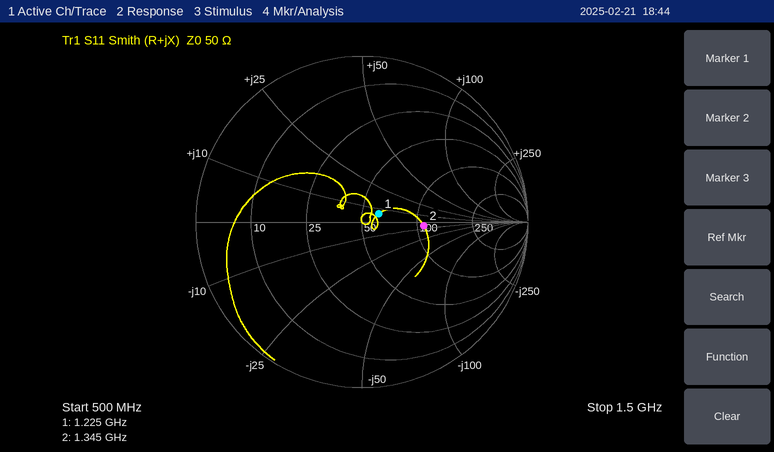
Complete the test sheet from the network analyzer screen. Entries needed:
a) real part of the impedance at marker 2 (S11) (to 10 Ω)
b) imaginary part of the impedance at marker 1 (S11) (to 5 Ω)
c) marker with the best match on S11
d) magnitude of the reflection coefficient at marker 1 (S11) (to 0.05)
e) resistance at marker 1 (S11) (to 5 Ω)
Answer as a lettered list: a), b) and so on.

a) 110 Ω
b) +5 Ω
c) marker 1
d) 0.10
e) 60 Ω
